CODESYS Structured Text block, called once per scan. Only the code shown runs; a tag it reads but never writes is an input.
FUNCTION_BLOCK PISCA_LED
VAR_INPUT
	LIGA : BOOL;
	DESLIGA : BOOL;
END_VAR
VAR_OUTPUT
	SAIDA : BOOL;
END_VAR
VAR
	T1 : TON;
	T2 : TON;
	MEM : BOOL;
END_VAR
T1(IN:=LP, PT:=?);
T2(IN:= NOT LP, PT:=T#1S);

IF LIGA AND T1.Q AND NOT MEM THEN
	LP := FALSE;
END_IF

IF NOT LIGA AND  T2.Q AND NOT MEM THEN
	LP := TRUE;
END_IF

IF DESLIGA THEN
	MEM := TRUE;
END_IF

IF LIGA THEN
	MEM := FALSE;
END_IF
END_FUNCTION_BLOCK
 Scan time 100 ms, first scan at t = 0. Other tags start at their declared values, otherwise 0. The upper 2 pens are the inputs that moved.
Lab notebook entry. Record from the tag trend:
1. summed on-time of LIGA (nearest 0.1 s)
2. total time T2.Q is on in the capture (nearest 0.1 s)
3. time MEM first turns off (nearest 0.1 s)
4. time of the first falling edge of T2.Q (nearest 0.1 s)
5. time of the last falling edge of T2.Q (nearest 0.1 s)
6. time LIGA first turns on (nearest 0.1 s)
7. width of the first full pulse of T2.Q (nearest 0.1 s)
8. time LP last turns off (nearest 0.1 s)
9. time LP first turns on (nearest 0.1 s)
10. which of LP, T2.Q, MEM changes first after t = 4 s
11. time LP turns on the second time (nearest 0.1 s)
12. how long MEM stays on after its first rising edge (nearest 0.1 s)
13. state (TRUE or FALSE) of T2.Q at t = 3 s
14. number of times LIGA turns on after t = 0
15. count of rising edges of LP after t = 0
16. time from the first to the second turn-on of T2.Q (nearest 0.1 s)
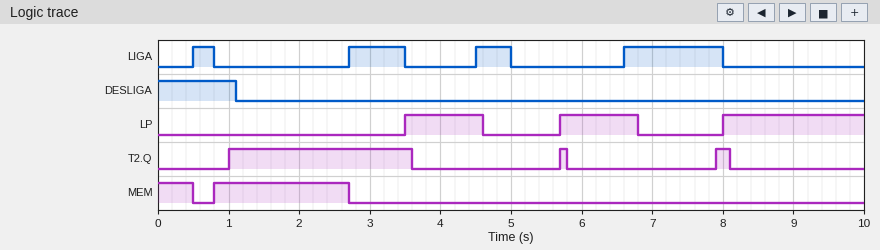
3.0 s
2.9 s
0.5 s
3.6 s
8.1 s
0.5 s
2.6 s
6.8 s
3.5 s
LP
5.7 s
1.9 s
TRUE
4
3
4.7 s
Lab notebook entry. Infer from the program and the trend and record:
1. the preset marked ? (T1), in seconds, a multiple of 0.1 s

1.0 s
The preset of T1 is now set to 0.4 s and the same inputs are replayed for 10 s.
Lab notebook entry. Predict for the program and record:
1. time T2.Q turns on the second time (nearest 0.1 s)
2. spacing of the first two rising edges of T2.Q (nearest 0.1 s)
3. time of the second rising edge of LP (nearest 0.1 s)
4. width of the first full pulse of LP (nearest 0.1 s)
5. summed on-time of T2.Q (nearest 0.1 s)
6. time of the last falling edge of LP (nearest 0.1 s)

5.6 s
4.6 s
5.6 s
1.0 s
3.1 s
6.6 s
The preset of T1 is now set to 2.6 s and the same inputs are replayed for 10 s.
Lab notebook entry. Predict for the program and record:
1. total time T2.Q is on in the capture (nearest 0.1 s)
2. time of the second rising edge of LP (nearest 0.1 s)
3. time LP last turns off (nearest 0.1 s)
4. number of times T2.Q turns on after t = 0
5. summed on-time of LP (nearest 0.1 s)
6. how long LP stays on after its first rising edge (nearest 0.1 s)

3.0 s
8.0 s
6.6 s
2
5.1 s
3.1 s
